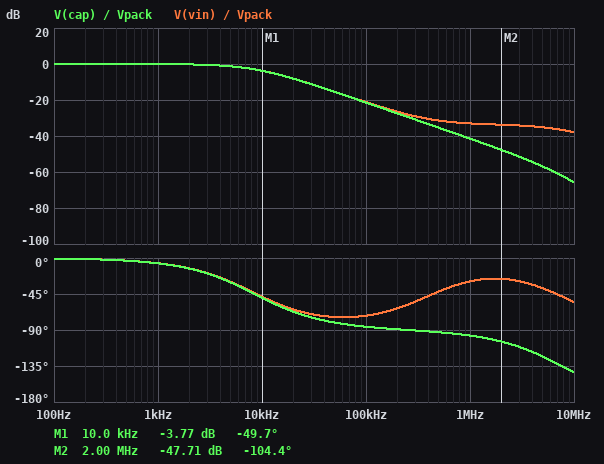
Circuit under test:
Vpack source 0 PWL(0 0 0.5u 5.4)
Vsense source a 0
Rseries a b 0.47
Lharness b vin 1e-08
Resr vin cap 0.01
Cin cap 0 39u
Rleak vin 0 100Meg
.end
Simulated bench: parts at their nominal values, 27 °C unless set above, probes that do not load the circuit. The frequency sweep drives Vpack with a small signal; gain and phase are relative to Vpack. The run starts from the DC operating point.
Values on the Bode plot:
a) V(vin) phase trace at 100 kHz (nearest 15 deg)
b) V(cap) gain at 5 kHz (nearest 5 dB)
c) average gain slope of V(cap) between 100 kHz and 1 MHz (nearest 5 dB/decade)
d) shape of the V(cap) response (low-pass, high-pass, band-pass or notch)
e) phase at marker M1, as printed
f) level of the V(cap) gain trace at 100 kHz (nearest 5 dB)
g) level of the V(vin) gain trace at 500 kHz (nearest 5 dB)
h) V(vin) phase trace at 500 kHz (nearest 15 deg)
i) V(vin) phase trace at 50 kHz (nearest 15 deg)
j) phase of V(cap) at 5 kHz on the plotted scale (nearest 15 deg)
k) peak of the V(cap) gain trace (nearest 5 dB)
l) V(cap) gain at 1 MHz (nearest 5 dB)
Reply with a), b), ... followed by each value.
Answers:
a) -75 deg
b) 0 dB
c) -20 dB/decade
d) low-pass
e) -49.7 deg
f) -20 dB
g) -30 dB
h) -45 deg
i) -75 deg
j) -30 deg
k) 0 dB
l) -40 dB
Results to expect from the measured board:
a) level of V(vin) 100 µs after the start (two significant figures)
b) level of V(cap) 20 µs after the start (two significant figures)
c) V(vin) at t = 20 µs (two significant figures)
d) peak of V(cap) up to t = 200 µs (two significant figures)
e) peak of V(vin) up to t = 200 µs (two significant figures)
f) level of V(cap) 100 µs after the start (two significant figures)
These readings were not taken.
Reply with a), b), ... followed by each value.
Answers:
a) 5.4 V
b) 3.5 V
c) 3.6 V
d) 5.4 V
e) 5.4 V
f) 5.4 V
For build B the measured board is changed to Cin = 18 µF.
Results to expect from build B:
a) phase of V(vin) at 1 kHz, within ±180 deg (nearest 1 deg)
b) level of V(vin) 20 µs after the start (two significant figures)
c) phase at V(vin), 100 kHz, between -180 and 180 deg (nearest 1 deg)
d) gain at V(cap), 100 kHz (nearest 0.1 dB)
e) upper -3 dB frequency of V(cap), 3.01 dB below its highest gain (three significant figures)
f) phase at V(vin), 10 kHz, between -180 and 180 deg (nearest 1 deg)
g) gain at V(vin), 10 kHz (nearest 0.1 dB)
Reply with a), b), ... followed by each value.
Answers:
a) -3 deg
b) 4.9 V
c) -74 deg
d) -14.8 dB
e) 18.5 kHz
f) -28 deg
g) -1.1 dB
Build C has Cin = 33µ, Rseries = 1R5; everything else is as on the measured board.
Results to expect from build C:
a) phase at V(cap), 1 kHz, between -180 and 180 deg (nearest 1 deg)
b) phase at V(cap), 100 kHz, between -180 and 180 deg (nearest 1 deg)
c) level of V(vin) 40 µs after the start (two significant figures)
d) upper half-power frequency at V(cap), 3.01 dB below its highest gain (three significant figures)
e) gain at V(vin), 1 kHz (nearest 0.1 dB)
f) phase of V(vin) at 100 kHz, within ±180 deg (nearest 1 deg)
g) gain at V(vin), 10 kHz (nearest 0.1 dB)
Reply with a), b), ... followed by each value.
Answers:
a) -17 deg
b) -88 deg
c) 3.0 V
d) 3.19 kHz
e) -0.4 dB
f) -77 deg
g) -10.3 dB
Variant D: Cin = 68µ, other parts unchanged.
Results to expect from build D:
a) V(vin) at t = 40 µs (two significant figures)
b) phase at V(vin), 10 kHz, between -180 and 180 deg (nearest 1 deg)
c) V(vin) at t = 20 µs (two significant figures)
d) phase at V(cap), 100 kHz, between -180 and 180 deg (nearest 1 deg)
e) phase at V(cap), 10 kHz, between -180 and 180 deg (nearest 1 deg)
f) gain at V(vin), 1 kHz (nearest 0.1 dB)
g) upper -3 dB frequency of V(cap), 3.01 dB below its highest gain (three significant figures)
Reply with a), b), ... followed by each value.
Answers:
a) 3.8 V
b) -62 deg
c) 2.5 V
d) -88 deg
e) -64 deg
f) -0.2 dB
g) 4.88 kHz
